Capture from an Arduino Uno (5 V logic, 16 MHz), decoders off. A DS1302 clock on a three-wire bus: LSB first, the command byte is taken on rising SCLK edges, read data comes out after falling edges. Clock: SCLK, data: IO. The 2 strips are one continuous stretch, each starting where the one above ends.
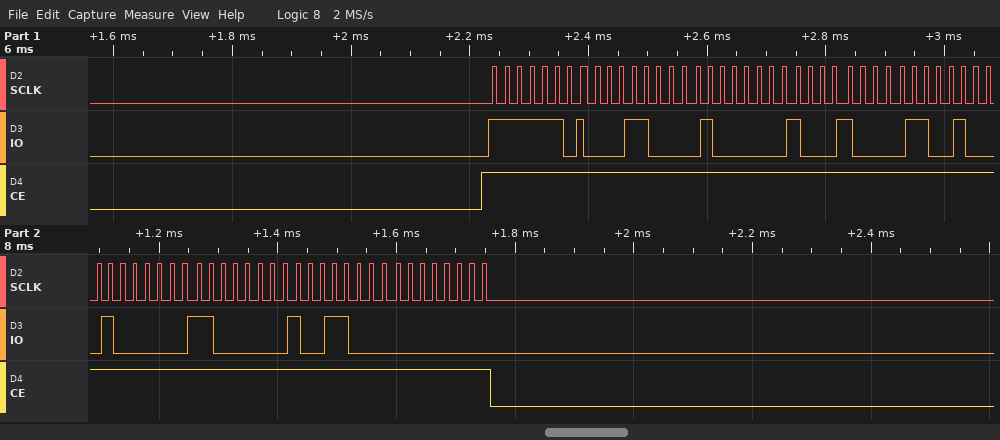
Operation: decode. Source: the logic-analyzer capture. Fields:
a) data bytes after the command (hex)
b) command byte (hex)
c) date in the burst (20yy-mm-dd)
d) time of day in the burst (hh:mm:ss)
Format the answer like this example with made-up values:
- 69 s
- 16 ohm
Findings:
- 18 02 11 26 02 03 19 00
- 0xBF
- 2019-02-26
- 11:02:18
